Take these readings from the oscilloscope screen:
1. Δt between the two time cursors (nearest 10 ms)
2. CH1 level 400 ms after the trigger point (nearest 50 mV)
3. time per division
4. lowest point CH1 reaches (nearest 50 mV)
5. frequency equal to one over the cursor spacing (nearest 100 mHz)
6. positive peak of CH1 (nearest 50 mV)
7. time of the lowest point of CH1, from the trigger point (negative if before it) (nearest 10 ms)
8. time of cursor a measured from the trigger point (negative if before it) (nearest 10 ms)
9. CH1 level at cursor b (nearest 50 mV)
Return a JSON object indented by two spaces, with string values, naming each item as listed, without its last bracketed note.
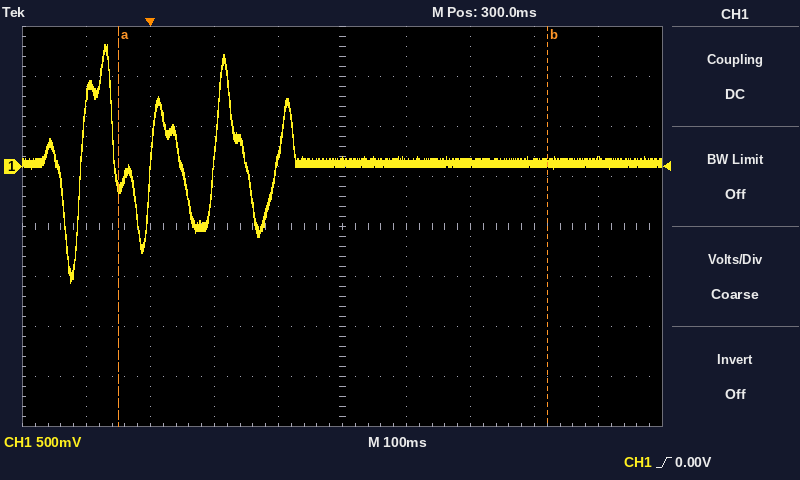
{
  "Δt between the two time cursors": "670 ms",
  "CH1 level 400 ms after the trigger point": "50 mV",
  "time per division": "100 ms",
  "lowest point CH1 reaches": "-1.15 V",
  "frequency equal to one over the cursor spacing": "1.5 Hz",
  "positive peak of CH1": "1.20 V",
  "time of the lowest point of CH1, from the trigger point (negative if before it)": "-120 ms",
  "time of cursor a measured from the trigger point (negative if before it)": "-50 ms",
  "CH1 level at cursor b": "50 mV"
}
